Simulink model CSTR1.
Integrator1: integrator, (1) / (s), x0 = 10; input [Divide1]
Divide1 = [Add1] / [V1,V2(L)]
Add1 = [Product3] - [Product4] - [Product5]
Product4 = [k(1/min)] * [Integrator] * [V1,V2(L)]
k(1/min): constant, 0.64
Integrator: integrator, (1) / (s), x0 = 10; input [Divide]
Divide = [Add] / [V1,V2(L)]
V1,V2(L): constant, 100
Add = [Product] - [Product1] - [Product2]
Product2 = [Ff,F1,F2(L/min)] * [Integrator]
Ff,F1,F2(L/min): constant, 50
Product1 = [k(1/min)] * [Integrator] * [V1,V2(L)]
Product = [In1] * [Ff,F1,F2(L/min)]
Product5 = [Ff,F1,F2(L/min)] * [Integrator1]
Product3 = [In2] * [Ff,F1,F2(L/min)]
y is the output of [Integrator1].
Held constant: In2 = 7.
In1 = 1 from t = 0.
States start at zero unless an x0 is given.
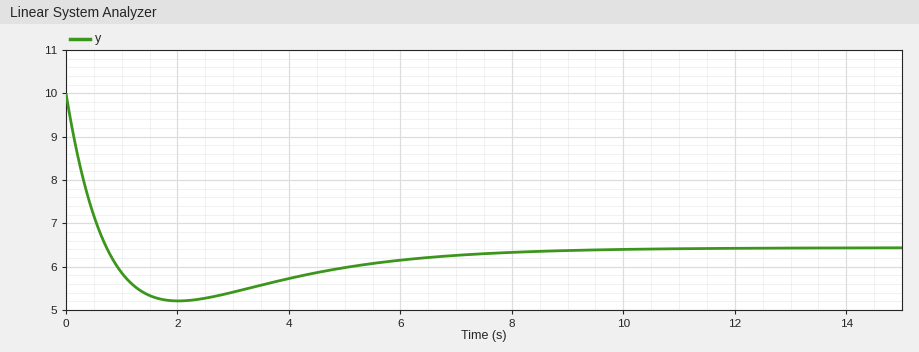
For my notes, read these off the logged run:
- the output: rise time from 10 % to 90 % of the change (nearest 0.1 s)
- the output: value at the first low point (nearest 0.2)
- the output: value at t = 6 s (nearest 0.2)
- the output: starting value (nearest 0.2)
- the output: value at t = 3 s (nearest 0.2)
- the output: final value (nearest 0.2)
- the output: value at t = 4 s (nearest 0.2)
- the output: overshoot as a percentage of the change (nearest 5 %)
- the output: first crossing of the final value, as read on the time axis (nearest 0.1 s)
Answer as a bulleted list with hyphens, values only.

- 0.6 s
- 5.2
- 6.2
- 10.0
- 5.4
- 6.4
- 5.8
- 35 %
- 0.7 s
